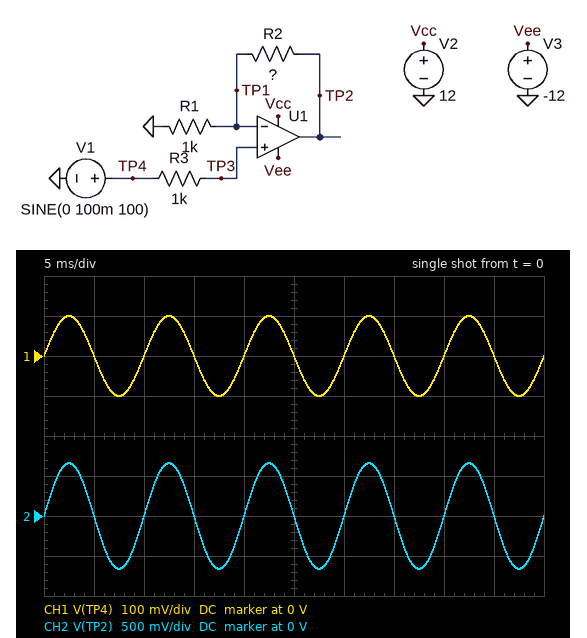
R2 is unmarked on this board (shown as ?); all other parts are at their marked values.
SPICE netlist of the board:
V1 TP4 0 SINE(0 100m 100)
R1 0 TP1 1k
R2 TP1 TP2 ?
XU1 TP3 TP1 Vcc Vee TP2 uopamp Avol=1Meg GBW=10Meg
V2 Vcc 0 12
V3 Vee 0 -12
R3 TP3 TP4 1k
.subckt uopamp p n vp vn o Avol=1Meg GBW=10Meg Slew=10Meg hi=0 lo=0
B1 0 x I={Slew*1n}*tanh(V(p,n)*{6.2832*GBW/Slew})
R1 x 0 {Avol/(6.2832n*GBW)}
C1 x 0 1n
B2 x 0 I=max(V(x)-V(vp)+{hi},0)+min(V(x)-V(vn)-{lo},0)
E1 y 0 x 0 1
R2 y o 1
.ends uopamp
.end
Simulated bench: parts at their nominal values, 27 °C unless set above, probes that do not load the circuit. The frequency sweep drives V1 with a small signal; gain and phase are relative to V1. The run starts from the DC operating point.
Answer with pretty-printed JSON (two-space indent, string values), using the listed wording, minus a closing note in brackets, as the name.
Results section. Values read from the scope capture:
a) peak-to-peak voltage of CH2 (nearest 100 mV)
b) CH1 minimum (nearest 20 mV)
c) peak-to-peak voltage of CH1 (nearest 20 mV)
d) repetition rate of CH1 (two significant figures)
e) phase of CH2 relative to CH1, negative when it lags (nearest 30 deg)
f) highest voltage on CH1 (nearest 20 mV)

{
  "peak-to-peak voltage of CH2": "1.3 V",
  "CH1 minimum": "-100 mV",
  "peak-to-peak voltage of CH1": "200 mV",
  "repetition rate of CH1": "100 Hz",
  "phase of CH2 relative to CH1, negative when it lags": "0 deg",
  "highest voltage on CH1": "100 mV"
}
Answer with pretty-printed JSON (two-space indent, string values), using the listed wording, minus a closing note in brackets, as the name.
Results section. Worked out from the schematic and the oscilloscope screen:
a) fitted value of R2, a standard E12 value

{
  "fitted value of R2, a standard E12 value": "5.6 kΩ"
}
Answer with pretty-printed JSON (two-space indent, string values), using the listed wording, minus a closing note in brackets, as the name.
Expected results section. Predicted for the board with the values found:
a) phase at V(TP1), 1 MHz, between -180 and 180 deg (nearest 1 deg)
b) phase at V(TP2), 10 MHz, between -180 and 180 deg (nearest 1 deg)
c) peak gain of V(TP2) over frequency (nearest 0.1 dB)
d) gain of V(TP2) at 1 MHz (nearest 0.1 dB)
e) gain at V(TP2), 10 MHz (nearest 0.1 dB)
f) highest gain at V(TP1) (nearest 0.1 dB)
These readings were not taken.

{
  "phase at V(TP1), 1 MHz, between -180 and 180 deg": "-33 deg",
  "phase at V(TP2), 10 MHz, between -180 and 180 deg": "-81 deg",
  "peak gain of V(TP2) over frequency": "16.4 dB",
  "gain of V(TP2) at 1 MHz": "14.8 dB",
  "gain at V(TP2), 10 MHz": "-0.1 dB",
  "highest gain at V(TP1)": "0 dB"
}
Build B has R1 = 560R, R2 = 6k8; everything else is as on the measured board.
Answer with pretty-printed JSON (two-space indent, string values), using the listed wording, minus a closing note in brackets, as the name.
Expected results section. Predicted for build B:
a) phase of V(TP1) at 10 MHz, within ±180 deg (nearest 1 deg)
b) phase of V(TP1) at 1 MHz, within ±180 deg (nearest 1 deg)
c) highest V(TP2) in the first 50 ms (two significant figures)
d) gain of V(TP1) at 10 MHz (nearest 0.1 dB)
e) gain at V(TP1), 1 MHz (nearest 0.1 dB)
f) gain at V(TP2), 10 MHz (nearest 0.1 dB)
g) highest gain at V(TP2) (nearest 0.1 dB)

{
  "phase of V(TP1) at 10 MHz, within ±180 deg": "-86 deg",
  "phase of V(TP1) at 1 MHz, within ±180 deg": "-53 deg",
  "highest V(TP2) in the first 50 ms": "1.3 V",
  "gain of V(TP1) at 10 MHz": "-22.4 dB",
  "gain at V(TP1), 1 MHz": "-4.4 dB",
  "gain at V(TP2), 10 MHz": "0 dB",
  "highest gain at V(TP2)": "22.4 dB"
}
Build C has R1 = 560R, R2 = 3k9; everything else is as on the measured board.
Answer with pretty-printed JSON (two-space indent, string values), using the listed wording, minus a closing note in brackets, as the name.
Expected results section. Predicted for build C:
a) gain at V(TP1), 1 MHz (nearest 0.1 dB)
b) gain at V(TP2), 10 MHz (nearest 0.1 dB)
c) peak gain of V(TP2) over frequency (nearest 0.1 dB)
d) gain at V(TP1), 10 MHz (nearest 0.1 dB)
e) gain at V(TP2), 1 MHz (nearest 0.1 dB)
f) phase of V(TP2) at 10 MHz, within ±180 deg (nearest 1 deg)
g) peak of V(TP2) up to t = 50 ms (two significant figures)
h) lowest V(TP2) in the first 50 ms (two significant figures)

{
  "gain at V(TP1), 1 MHz": "-2.1 dB",
  "gain at V(TP2), 10 MHz": "-0.1 dB",
  "peak gain of V(TP2) over frequency": "18.0 dB",
  "gain at V(TP1), 10 MHz": "-18.1 dB",
  "gain at V(TP2), 1 MHz": "15.9 dB",
  "phase of V(TP2) at 10 MHz, within ±180 deg": "-83 deg",
  "peak of V(TP2) up to t = 50 ms": "800 mV",
  "lowest V(TP2) in the first 50 ms": "-800 mV"
}
